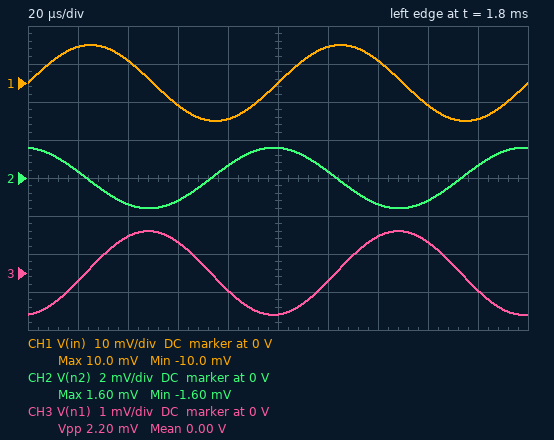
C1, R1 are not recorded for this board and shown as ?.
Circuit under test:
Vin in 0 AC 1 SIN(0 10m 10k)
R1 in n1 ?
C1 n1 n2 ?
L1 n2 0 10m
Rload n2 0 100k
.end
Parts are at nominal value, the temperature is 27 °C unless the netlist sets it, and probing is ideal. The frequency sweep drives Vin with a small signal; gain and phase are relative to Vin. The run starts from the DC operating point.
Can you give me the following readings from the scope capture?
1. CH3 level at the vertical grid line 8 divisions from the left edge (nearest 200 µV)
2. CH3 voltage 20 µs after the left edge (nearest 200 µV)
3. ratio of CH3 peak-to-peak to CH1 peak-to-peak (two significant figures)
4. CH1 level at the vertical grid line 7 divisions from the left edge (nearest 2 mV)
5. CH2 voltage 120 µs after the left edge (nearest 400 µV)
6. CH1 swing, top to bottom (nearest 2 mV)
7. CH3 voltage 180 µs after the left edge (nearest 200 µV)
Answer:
800 µV
-200 µV
0.11
6 mV
400 µV
20 mV
-400 µV
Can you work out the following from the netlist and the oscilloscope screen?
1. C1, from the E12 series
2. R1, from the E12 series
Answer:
15 nF
3.9 kΩ
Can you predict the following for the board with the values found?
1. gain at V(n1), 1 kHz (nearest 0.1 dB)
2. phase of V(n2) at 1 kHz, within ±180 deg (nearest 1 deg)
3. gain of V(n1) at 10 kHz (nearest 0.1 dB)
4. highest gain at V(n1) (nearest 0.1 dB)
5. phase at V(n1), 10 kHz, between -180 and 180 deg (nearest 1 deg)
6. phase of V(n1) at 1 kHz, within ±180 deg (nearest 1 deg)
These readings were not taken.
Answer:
-0.6 dB
160 deg
-19.2 dB
0 dB
-83 deg
-20 deg
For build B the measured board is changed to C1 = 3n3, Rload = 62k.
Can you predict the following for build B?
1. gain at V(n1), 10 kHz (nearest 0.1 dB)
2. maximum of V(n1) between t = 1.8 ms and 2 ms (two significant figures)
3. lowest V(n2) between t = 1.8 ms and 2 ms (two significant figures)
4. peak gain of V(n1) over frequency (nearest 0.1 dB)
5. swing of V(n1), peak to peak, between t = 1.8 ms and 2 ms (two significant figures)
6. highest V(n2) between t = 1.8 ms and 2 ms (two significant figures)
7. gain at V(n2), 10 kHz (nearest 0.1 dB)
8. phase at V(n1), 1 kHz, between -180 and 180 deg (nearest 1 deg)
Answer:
-2.7 dB
7.3 mV
-1.1 mV
0 dB
15 mV
1.1 mV
-19.2 dB
-5 deg
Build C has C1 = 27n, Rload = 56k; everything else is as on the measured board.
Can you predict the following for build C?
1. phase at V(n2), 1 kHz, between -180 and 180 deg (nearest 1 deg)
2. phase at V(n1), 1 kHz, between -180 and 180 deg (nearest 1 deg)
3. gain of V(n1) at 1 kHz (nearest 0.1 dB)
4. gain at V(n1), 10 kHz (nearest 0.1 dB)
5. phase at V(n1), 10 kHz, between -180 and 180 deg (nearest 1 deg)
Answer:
146 deg
-34 deg
-1.6 dB
-39.9 dB
79 deg
